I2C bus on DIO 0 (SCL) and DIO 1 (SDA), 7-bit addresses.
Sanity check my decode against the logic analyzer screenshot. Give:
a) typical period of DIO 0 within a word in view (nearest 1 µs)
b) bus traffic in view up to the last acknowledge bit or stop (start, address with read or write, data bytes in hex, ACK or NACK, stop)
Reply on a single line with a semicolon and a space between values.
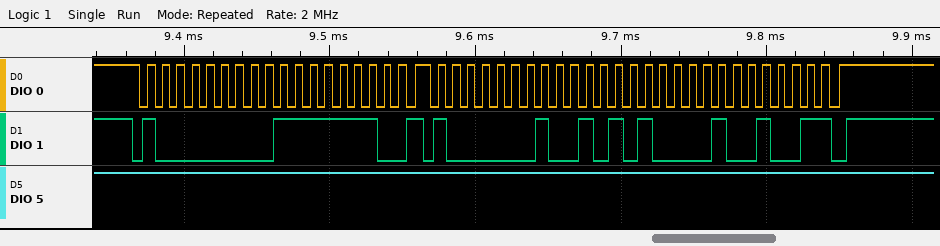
10 µs; start, address 40 write ACK, FE ACK, repeated start, address 40 read ACK, 54 ACK, 49 NACK, stop
